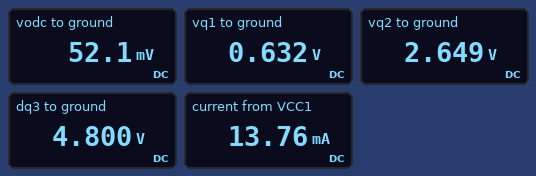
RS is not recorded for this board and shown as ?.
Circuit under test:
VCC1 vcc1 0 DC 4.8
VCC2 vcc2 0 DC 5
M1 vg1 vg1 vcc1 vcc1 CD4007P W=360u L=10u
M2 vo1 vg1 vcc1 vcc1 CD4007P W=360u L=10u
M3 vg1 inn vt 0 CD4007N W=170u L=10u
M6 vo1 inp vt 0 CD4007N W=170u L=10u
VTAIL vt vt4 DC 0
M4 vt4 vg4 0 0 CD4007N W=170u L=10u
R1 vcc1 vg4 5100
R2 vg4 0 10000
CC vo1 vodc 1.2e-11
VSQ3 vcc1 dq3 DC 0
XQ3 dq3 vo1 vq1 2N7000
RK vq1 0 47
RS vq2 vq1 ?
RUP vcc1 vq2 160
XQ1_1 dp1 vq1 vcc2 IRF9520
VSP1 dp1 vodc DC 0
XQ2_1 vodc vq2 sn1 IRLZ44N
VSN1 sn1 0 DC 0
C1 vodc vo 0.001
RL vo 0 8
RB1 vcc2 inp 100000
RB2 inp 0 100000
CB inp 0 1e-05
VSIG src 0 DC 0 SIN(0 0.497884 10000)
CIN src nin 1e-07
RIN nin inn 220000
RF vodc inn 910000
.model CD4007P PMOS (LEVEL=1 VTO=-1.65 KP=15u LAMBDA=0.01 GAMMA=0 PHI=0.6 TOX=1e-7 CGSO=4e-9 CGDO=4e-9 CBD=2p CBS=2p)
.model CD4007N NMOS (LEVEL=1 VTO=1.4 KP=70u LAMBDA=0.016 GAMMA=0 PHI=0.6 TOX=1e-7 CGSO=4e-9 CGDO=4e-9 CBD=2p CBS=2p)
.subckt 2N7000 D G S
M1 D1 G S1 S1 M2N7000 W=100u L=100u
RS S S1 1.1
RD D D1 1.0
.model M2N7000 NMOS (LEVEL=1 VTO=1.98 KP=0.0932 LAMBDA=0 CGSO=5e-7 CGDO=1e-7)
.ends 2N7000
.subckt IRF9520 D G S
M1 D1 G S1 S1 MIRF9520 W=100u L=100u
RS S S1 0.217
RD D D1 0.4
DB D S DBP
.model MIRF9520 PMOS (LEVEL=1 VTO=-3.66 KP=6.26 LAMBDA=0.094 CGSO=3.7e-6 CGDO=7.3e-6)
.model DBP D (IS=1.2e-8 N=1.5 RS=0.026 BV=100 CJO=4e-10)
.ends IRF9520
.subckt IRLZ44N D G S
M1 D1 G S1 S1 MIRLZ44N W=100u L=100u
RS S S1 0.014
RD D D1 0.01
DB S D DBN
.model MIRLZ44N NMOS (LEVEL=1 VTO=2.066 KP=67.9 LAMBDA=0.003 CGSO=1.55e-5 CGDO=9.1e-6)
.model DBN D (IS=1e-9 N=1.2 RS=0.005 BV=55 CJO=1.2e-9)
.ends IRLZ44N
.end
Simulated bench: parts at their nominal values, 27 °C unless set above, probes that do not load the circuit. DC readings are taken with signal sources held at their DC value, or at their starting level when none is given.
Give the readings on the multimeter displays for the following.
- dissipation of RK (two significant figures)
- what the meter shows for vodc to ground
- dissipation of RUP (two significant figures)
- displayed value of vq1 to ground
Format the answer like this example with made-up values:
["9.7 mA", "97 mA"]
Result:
["8.5 mW", "52.1 mV", "29 mW", "0.632 V"]
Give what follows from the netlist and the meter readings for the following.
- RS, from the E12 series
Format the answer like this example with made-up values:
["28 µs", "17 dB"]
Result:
["150 Ω"]
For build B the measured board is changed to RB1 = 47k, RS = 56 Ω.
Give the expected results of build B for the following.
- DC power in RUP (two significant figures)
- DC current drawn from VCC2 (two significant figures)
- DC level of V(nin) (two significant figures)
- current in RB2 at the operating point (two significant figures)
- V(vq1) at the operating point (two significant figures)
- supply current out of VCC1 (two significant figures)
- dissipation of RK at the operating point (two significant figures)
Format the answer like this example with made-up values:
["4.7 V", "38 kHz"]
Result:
["45 mW", "77 mA", "3.8 V", "34 µA", "1.2 V", "27 mA", "29 mW"]
